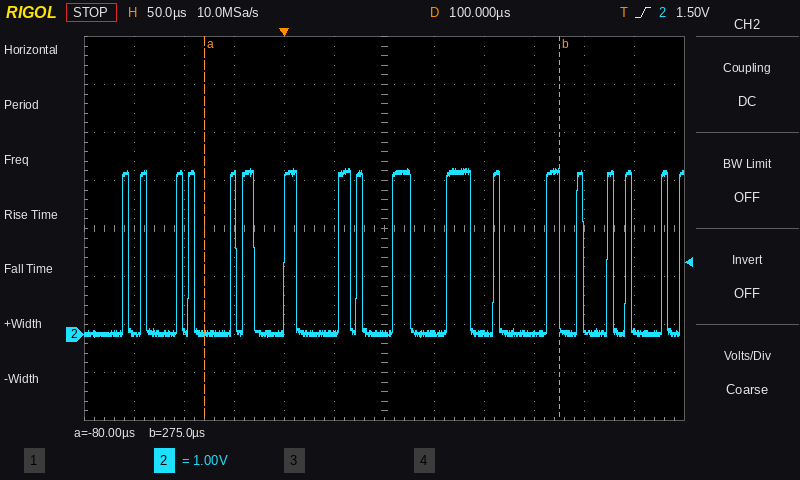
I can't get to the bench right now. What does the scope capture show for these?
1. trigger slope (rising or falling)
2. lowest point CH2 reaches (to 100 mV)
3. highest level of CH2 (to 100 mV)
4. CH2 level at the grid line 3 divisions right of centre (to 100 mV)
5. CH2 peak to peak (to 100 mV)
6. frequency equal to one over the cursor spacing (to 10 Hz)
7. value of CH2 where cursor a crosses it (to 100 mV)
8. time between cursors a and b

rising
-100 mV
3.4 V
0.0 V
3.5 V
2.82 kHz
0.0 V
355 µs
